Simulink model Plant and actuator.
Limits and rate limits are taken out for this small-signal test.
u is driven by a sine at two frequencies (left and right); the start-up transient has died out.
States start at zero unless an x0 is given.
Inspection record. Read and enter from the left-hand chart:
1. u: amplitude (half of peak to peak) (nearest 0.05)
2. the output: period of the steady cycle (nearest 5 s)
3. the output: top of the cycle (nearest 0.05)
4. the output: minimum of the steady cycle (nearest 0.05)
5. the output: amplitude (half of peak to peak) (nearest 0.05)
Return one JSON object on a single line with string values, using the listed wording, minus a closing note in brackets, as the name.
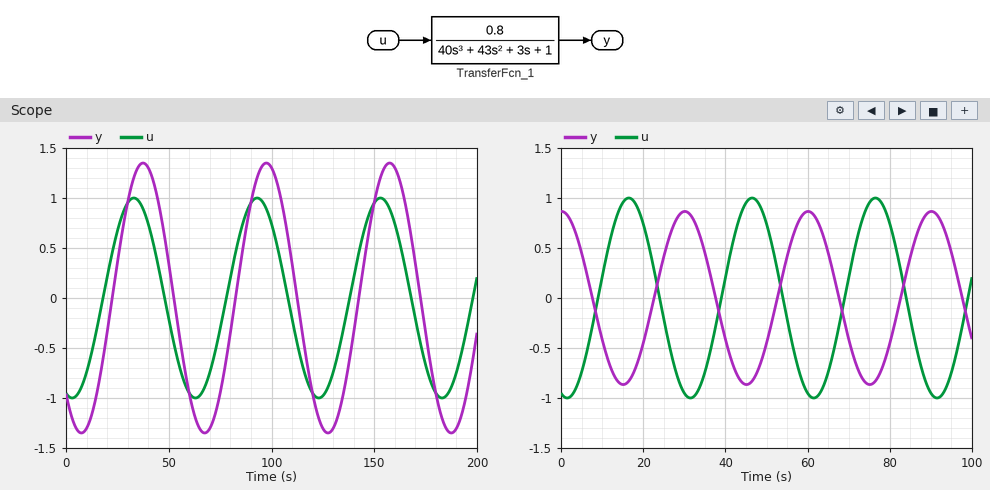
{"u: amplitude (half of peak to peak)": "1.00", "the output: period of the steady cycle": "60 s", "the output: top of the cycle": "1.35", "the output: minimum of the steady cycle": "-1.35", "the output: amplitude (half of peak to peak)": "1.35"}
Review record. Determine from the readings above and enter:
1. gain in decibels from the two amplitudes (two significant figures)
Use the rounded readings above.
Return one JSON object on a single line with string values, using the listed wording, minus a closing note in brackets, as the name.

{"gain in decibels from the two amplitudes": "2.6 dB"}
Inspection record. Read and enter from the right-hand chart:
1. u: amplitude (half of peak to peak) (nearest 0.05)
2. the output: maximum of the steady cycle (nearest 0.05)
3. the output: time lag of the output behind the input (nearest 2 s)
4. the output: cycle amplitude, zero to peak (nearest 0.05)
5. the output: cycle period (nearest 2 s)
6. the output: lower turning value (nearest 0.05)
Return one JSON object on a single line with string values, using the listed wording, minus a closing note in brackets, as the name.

{"u: amplitude (half of peak to peak)": "1.00", "the output: maximum of the steady cycle": "0.85", "the output: time lag of the output behind the input": "14 s", "the output: cycle amplitude, zero to peak": "0.85", "the output: cycle period": "30 s", "the output: lower turning value": "-0.85"}
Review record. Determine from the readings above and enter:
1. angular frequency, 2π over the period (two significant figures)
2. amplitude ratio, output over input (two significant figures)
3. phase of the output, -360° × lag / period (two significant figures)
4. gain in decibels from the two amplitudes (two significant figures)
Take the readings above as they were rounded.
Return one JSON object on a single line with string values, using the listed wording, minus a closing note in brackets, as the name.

{"angular frequency, 2π over the period": "0.21 rad/s", "amplitude ratio, output over input": "0.85", "phase of the output, -360° × lag / period": "-170°", "gain in decibels from the two amplitudes": "-1.4 dB"}
